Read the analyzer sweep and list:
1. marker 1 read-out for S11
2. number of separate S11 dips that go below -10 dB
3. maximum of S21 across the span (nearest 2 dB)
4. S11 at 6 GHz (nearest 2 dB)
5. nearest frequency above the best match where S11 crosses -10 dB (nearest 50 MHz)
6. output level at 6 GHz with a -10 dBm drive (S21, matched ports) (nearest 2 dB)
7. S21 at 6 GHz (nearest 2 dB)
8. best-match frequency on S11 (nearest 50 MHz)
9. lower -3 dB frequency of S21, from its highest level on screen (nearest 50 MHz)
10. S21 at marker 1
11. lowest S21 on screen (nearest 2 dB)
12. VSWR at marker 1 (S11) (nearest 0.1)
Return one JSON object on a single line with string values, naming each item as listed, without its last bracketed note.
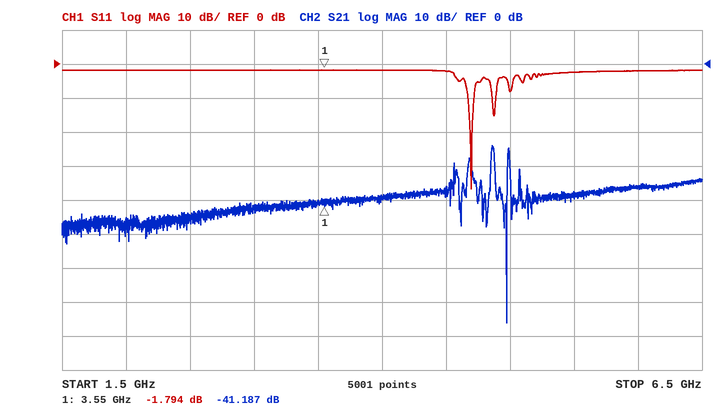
{"marker 1 read-out for S11": "-1.794 dB", "number of separate S11 dips that go below -10 dB": "2", "maximum of S21 across the span": "-24 dB", "S11 at 6 GHz": "-2 dB", "nearest frequency above the best match where S11 crosses -10 dB": "4.70 GHz", "output level at 6 GHz with a -10 dBm drive (S21, matched ports)": "-46 dBm", "S21 at 6 GHz": "-36 dB", "best-match frequency on S11": "4.70 GHz", "lower -3 dB frequency of S21, from its highest level on screen": "4.85 GHz", "S21 at marker 1": "-41.187 dB", "lowest S21 on screen": "-76 dB", "VSWR at marker 1 (S11)": "9.7"}
